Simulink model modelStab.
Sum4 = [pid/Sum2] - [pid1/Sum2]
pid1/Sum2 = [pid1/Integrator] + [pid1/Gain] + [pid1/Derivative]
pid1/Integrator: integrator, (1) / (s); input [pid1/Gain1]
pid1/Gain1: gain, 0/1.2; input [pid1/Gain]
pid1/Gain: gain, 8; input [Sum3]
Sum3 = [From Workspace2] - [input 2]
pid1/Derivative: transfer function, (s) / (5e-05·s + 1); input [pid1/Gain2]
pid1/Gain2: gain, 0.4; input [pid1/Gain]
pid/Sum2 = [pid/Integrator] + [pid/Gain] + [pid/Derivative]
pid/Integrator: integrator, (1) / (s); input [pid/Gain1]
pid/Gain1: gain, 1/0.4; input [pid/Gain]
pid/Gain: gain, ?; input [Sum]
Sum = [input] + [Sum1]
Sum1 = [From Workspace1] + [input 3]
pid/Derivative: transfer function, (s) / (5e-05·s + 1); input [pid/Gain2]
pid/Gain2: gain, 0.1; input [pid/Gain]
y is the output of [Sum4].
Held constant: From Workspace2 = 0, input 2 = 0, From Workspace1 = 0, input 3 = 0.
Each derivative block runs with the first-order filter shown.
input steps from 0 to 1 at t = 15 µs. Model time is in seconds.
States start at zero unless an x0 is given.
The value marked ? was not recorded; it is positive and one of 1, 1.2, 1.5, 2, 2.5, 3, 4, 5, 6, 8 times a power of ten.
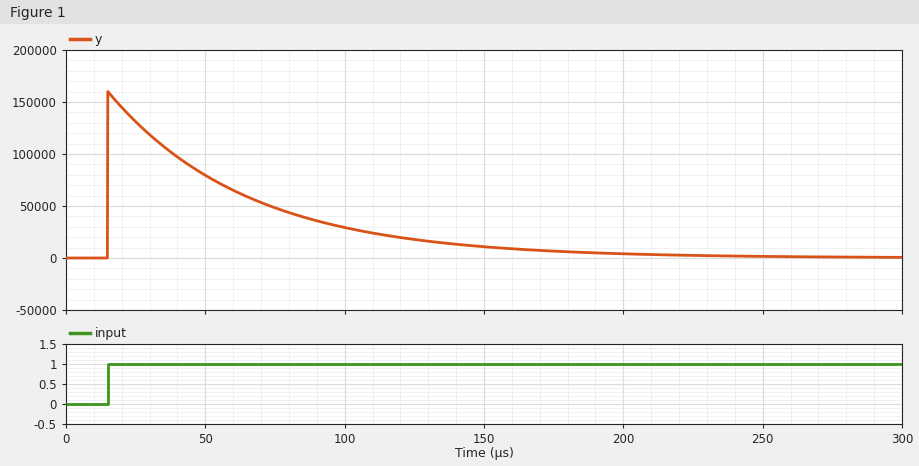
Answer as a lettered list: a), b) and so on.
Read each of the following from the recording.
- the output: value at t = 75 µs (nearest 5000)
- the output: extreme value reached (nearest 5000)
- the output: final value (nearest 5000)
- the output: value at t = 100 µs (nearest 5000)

a) 50000
b) 160000
c) 0
d) 30000
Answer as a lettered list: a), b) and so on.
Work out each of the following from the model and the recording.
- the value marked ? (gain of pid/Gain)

a) 80
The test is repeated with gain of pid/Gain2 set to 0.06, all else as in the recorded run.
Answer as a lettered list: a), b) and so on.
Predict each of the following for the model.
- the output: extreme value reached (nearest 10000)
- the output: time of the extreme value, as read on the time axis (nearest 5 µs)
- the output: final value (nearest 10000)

a) 100000
b) 15 µs
c) 0
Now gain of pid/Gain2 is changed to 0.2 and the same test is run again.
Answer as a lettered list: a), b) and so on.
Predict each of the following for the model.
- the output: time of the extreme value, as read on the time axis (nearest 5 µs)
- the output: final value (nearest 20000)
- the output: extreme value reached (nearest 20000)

a) 15 µs
b) 0
c) 320000
